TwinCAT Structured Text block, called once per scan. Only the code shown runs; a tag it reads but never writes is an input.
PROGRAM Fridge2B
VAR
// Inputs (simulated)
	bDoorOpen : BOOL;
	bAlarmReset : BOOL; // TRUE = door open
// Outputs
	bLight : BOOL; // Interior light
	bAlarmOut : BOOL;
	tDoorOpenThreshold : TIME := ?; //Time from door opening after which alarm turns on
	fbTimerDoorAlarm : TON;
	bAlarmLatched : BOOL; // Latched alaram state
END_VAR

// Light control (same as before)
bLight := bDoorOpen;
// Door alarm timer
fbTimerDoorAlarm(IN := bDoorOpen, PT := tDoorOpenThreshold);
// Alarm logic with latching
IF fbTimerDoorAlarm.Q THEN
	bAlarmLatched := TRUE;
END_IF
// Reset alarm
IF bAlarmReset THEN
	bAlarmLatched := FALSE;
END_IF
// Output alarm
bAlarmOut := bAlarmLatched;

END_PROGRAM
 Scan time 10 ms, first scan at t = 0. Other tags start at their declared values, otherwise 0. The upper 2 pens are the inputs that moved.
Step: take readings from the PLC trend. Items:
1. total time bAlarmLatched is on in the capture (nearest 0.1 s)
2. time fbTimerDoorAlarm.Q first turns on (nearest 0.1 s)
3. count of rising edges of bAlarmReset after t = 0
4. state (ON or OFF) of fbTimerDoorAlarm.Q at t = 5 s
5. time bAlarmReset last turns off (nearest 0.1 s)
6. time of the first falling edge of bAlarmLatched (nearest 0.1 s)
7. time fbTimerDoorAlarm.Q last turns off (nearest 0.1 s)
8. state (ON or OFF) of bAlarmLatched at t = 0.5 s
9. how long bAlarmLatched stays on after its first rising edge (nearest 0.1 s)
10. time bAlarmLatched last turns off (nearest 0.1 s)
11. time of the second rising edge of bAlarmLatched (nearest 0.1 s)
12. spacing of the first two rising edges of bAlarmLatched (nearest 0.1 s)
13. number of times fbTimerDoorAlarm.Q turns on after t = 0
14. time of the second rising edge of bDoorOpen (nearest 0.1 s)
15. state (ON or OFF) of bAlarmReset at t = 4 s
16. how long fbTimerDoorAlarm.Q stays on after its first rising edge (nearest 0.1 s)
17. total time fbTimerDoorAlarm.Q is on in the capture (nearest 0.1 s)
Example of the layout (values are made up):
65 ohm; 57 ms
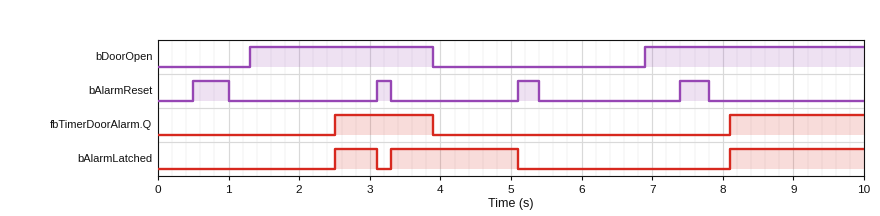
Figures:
4.3 s; 2.5 s; 4; OFF; 7.8 s; 3.1 s; 3.9 s; OFF; 0.6 s; 5.1 s; 3.3 s; 0.8 s; 2; 6.9 s; OFF; 1.4 s; 3.3 s
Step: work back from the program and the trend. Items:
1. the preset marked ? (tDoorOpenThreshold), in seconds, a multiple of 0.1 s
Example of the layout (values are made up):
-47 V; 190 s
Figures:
1.2 s
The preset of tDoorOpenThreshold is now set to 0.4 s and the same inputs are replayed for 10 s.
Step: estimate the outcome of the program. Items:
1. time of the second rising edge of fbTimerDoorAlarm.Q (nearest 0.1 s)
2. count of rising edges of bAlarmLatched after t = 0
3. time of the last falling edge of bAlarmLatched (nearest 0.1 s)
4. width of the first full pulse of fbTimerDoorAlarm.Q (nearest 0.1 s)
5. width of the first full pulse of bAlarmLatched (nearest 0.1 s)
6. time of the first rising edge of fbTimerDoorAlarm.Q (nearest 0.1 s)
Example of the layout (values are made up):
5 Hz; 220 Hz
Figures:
7.3 s; 4; 7.4 s; 2.2 s; 1.4 s; 1.7 s
